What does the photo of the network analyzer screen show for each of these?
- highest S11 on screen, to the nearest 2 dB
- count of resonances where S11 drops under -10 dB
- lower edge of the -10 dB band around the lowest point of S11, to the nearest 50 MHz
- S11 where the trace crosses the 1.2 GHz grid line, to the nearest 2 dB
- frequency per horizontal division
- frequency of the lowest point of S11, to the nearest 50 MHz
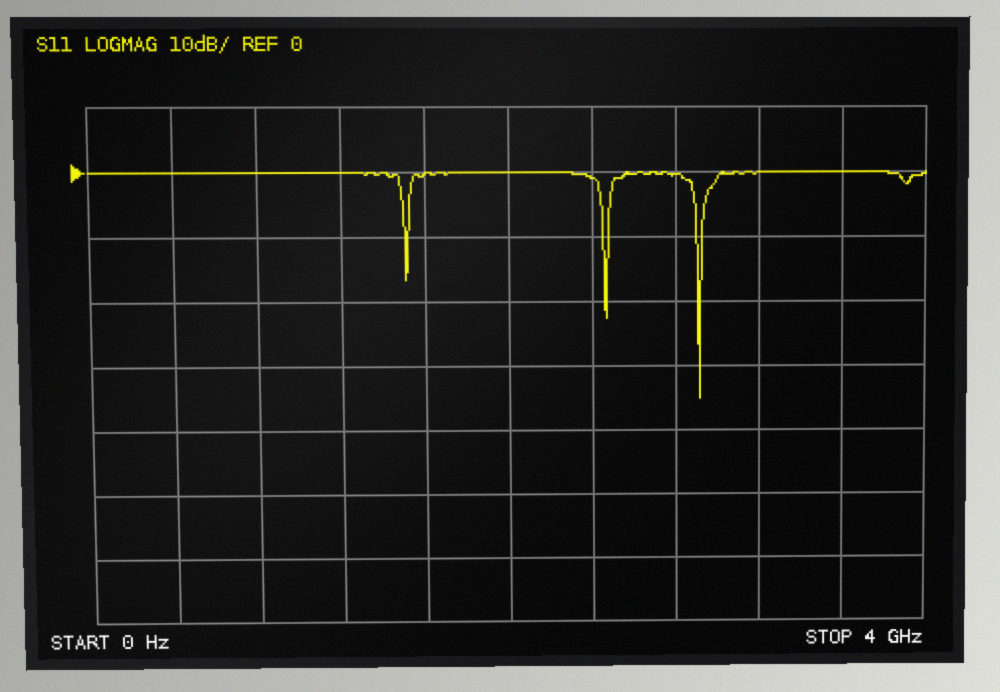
0 dB
3
2.90 GHz
0 dB
400 MHz
2.90 GHz
